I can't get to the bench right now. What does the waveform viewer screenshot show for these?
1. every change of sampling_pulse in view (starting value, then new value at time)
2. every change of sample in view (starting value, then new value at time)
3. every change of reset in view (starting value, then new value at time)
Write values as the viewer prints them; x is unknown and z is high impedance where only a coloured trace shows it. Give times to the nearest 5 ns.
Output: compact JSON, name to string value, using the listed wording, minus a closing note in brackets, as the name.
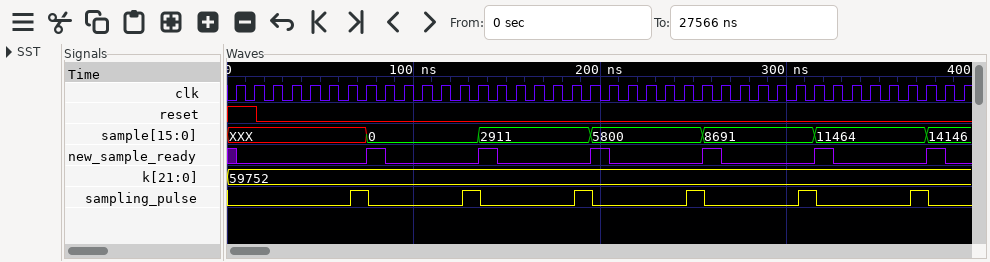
{"every change of sampling_pulse in view": "0, 1 at 65 ns, 0 at 75 ns, 1 at 125 ns, 0 at 135 ns, 1 at 185 ns, 0 at 195 ns, 1 at 245 ns, 0 at 255 ns, 1 at 305 ns, 0 at 315 ns, 1 at 365 ns, 0 at 375 ns", "every change of sample in view": "XXX, 0 at 75 ns, 2911 at 135 ns, 5800 at 195 ns, 8691 at 255 ns, 11464 at 315 ns, 14146 at 375 ns", "every change of reset in view": "1, 0 at 15 ns"}
